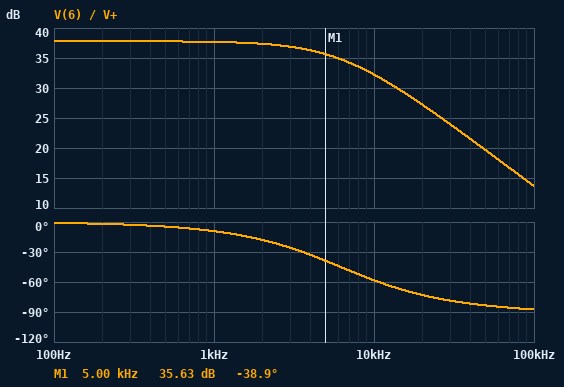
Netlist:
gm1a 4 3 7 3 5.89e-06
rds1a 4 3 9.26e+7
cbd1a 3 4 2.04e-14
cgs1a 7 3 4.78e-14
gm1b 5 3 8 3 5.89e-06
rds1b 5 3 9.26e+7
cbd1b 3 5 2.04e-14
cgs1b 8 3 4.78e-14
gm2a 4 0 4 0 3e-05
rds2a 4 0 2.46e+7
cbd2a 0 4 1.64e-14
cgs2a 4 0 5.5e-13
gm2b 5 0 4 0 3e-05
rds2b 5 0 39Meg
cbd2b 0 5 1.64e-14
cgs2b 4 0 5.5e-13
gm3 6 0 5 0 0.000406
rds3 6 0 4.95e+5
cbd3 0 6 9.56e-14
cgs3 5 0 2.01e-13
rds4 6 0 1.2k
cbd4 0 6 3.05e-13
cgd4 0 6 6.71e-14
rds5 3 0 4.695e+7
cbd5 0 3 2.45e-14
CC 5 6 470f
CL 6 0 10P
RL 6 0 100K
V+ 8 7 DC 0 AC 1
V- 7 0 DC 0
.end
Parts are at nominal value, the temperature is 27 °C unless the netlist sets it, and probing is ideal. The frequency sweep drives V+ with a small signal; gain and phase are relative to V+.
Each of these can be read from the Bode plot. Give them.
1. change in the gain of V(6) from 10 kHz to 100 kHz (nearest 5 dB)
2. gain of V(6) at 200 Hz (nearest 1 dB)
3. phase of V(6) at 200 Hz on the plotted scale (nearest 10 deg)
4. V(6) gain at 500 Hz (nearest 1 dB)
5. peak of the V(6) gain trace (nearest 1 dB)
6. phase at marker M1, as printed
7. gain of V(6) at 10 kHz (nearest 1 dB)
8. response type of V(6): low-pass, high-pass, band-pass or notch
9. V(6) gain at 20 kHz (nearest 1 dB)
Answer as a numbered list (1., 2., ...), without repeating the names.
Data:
1. -20 dB
2. 38 dB
3. 0 deg
4. 38 dB
5. 38 dB
6. -38.9 deg
7. 32 dB
8. low-pass
9. 27 dB
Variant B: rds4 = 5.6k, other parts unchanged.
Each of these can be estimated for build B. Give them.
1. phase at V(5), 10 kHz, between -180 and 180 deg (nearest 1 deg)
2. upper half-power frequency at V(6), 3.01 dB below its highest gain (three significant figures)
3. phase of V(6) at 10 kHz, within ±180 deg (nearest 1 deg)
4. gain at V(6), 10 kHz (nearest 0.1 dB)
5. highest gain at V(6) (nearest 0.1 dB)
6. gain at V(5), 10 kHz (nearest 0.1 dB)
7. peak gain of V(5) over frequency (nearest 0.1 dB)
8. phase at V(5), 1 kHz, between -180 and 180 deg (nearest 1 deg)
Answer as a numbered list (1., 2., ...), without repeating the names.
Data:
1. 109 deg
2. 3.39 kHz
3. -71 deg
4. 40.9 dB
5. 50.7 dB
6. 34.3 dB
7. 44.2 dB
8. 164 deg
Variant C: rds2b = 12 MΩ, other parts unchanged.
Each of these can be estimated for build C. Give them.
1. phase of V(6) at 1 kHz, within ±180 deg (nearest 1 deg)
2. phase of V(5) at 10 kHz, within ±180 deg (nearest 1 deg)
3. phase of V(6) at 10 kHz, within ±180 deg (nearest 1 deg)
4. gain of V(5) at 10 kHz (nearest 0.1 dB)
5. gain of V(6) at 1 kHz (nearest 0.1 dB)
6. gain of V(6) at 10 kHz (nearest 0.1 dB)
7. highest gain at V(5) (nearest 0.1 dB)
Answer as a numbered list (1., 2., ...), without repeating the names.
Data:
1. -4 deg
2. 148 deg
3. -32 deg
4. 34.5 dB
5. 29.5 dB
6. 28.1 dB
7. 35.9 dB
